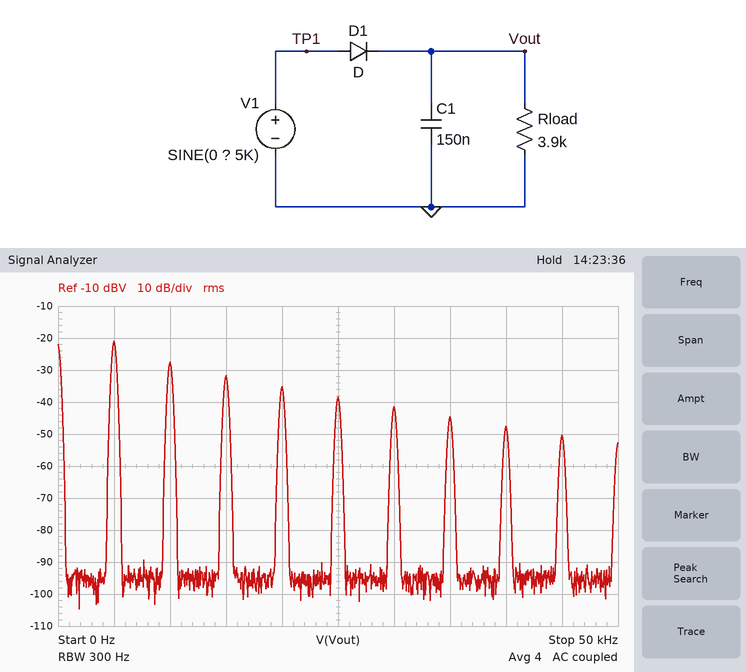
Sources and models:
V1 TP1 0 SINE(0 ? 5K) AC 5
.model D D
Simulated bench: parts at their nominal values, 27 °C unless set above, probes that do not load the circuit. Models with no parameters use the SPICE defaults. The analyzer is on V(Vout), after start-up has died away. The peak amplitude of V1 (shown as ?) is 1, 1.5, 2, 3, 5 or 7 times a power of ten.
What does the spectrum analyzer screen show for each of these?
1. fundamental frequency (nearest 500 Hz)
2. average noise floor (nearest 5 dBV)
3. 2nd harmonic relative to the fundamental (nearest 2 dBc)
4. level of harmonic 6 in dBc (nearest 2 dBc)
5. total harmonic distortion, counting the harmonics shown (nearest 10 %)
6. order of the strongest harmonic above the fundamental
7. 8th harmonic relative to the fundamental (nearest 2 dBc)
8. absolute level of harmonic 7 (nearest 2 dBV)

5.0 kHz
-95 dBV
-6 dBc
-20 dBc
60 %
2
-26 dBc
-44 dBV
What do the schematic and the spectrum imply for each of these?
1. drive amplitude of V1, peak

2 V
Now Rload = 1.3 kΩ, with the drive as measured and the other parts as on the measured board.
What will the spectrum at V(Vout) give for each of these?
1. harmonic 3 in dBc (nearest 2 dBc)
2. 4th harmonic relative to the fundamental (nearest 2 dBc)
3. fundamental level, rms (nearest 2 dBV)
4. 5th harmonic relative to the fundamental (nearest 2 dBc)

-12 dBc
-16 dBc
-14 dBV
-22 dBc
